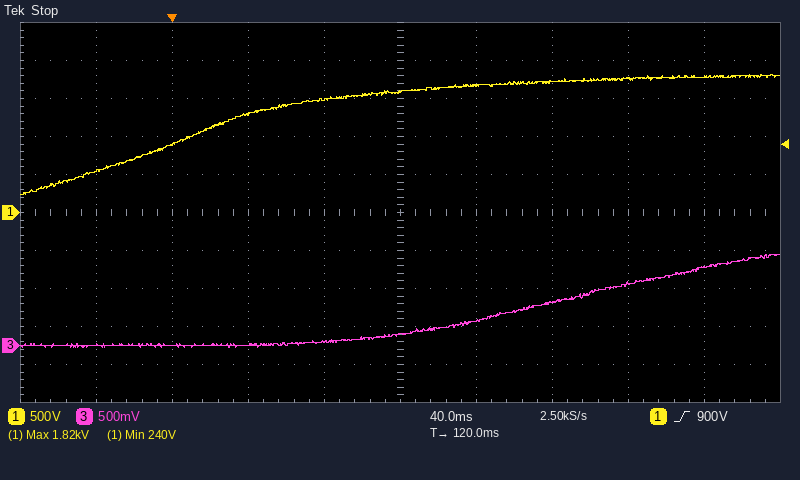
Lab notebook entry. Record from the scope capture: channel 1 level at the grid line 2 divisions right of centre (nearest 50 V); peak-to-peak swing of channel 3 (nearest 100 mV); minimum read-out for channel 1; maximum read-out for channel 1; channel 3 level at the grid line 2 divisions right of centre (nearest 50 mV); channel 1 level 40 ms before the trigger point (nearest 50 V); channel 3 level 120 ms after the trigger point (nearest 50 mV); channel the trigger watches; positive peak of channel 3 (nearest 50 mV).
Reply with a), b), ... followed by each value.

a) 1.70 kV
b) 1.20 V
c) 240 V
d) 1.82 kV
e) 550 mV
f) 550 V
g) 150 mV
h) channel 1
i) 1.20 V
